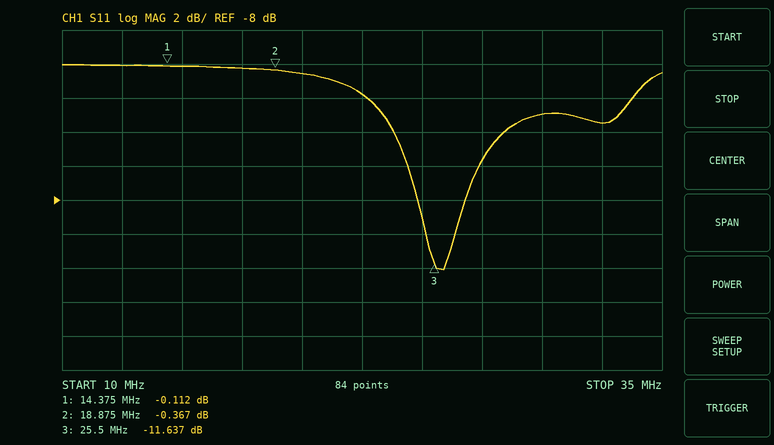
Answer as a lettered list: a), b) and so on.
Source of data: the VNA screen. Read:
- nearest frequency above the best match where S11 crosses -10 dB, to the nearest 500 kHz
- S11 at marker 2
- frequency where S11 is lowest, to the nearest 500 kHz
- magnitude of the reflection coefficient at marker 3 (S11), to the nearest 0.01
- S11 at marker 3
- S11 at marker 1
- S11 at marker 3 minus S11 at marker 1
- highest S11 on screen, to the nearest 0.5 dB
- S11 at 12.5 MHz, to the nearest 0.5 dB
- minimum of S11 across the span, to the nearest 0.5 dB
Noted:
a) 26.5 MHz
b) -0.367 dB
c) 26.0 MHz
d) 0.26
e) -11.637 dB
f) -0.112 dB
g) -11.525 dB
h) 0.0 dB
i) 0.0 dB
j) -12.0 dB
